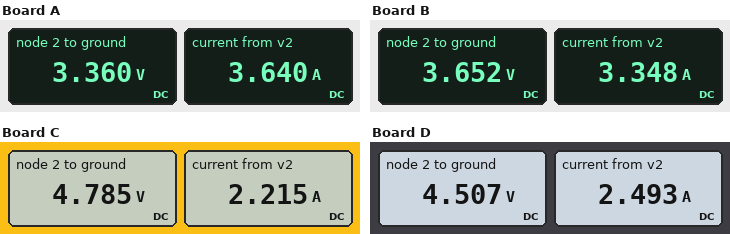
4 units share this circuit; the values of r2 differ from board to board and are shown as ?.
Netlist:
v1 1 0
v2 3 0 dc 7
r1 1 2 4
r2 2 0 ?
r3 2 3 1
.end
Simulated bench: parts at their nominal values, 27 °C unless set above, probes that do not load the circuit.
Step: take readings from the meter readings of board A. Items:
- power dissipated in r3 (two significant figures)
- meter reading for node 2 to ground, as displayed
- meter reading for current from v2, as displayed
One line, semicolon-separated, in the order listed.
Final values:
13 W; 3.360 V; 3.640 A
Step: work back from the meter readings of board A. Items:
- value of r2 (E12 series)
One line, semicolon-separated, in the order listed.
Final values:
1.2 Ω
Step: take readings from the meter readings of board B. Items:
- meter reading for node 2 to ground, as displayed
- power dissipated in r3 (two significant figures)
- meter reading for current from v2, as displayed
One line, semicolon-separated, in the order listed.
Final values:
3.652 V; 11 W; 3.348 A
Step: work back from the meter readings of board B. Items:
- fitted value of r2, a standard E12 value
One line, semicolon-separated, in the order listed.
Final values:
1.5 Ω
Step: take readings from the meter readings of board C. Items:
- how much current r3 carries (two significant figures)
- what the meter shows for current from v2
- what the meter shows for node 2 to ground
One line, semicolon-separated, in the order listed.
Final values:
2.2 A; 2.215 A; 4.785 V
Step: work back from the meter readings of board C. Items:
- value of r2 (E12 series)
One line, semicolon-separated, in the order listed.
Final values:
4.7 Ω
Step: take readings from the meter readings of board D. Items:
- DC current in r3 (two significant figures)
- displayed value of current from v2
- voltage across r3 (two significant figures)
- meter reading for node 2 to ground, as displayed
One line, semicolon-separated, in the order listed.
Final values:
2.5 A; 2.493 A; 2.5 V; 4.507 V
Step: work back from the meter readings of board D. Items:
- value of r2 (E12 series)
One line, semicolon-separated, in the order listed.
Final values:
3.3 Ω
